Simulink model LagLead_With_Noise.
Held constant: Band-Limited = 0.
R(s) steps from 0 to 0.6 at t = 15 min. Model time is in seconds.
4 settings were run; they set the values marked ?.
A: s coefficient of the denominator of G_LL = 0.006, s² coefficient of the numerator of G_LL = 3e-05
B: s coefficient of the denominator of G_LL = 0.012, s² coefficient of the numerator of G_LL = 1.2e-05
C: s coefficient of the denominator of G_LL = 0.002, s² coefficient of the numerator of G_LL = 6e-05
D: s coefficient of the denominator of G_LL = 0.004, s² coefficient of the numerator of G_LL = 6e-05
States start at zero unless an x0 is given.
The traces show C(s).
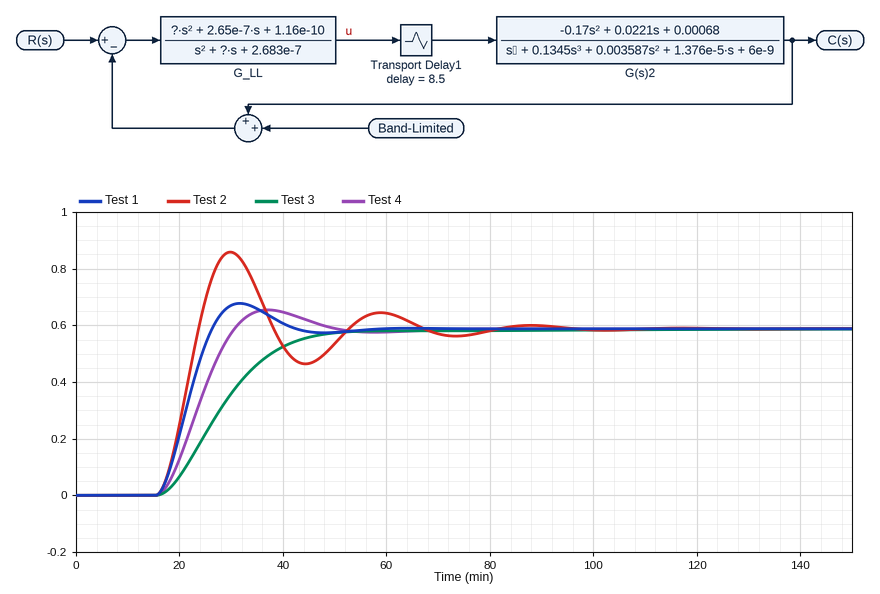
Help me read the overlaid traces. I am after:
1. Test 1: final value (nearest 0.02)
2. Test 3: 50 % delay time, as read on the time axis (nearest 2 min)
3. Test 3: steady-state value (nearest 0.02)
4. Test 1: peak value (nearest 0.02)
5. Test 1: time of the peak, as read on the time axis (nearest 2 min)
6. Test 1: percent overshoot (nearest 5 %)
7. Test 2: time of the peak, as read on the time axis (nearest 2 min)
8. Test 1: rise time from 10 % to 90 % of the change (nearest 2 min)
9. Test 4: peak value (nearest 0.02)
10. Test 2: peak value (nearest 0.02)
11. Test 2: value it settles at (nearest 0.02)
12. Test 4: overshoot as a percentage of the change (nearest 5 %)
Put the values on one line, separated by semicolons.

0.58; 28 min; 0.58; 0.68; 32 min; 15 %; 30 min; 8 min; 0.66; 0.86; 0.58; 10 %
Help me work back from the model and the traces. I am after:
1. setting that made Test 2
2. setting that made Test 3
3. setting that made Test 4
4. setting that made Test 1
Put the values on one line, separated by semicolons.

C; B; A; D
